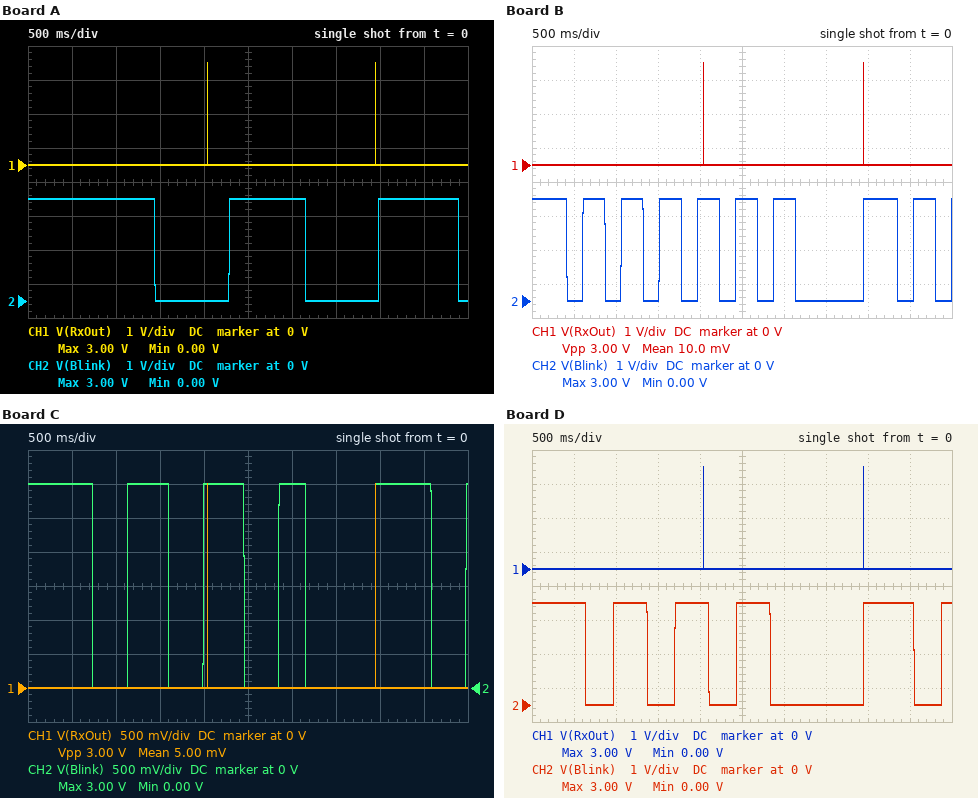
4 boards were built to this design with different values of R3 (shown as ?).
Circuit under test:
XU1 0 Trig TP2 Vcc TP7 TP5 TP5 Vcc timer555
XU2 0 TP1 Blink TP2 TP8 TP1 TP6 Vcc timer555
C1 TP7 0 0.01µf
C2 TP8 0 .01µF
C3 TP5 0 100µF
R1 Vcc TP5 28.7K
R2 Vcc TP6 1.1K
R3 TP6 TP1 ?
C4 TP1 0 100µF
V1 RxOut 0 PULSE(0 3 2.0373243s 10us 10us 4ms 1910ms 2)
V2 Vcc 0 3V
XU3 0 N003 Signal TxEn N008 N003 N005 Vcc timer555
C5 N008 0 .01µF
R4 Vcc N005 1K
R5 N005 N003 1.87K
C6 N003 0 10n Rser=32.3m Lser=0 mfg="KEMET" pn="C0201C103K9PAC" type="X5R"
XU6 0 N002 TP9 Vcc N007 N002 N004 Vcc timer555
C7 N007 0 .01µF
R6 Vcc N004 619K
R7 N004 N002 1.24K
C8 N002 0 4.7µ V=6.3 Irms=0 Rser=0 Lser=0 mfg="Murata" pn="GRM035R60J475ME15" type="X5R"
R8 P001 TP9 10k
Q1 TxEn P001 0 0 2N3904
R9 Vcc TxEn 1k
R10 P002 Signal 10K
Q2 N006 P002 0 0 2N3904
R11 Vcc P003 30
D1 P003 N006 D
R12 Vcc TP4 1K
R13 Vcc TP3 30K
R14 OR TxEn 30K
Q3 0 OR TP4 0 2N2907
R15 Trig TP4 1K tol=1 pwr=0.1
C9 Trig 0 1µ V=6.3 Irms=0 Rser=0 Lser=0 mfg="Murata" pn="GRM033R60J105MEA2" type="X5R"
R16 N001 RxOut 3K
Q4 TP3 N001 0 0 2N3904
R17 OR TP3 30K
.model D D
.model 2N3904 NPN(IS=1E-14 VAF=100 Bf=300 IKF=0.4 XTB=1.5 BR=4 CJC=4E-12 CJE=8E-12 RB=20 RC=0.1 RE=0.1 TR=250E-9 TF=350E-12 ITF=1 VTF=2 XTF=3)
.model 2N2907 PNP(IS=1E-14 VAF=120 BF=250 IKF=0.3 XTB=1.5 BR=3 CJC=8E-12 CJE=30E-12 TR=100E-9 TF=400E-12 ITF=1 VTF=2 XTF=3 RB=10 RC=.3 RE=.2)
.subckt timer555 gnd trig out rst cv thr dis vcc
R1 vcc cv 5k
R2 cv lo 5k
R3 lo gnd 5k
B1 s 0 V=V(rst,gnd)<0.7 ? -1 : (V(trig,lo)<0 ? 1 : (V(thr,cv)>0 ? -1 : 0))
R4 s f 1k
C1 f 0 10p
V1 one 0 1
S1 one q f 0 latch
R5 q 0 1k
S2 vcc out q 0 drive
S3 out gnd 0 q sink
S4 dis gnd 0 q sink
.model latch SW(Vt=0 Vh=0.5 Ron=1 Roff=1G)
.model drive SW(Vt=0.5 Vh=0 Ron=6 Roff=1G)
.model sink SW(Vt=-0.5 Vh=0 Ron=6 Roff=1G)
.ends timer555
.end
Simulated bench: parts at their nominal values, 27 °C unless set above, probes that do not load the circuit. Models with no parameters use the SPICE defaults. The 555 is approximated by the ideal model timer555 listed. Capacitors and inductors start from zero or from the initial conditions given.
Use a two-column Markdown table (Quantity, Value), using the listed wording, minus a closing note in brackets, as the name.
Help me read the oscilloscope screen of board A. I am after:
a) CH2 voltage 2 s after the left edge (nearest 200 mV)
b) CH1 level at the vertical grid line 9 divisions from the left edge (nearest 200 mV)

| Quantity | Value |
|---|---|
| CH2 voltage 2 s after the left edge | 0 V |
| CH1 level at the vertical grid line 9 divisions from the left edge | 0 V |
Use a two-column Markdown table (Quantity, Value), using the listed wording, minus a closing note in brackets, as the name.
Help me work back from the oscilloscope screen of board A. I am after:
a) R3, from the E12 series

| Quantity | Value |
|---|---|
| R3, from the E12 series | 12 kΩ |
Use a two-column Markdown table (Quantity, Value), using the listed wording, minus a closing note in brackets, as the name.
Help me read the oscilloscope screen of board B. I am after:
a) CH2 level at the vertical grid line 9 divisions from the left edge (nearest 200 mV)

| Quantity | Value |
|---|---|
| CH2 level at the vertical grid line 9 divisions from the left edge | 0 V |
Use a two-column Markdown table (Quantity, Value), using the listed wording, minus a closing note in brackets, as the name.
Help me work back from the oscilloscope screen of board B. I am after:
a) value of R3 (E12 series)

| Quantity | Value |
|---|---|
| value of R3 | 2.7 kΩ |
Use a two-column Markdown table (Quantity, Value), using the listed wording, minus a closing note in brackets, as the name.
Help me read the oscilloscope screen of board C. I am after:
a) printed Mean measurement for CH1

| Quantity | Value |
|---|---|
| printed Mean measurement for CH1 | 5.00 mV |
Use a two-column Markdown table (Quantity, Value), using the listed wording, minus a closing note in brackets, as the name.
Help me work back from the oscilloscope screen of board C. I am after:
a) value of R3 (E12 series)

| Quantity | Value |
|---|---|
| value of R3 | 5.6 kΩ |
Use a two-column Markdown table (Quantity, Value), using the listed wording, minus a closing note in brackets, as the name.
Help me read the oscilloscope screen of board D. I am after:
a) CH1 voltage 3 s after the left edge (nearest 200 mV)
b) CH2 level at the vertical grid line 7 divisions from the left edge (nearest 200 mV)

| Quantity | Value |
|---|---|
| CH1 voltage 3 s after the left edge | 0 V |
| CH2 level at the vertical grid line 7 divisions from the left edge | 0 V |
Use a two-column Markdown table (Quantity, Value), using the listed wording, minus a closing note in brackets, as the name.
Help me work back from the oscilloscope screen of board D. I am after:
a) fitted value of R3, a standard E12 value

| Quantity | Value |
|---|---|
| fitted value of R3, a standard E12 value | 4.7 kΩ |
